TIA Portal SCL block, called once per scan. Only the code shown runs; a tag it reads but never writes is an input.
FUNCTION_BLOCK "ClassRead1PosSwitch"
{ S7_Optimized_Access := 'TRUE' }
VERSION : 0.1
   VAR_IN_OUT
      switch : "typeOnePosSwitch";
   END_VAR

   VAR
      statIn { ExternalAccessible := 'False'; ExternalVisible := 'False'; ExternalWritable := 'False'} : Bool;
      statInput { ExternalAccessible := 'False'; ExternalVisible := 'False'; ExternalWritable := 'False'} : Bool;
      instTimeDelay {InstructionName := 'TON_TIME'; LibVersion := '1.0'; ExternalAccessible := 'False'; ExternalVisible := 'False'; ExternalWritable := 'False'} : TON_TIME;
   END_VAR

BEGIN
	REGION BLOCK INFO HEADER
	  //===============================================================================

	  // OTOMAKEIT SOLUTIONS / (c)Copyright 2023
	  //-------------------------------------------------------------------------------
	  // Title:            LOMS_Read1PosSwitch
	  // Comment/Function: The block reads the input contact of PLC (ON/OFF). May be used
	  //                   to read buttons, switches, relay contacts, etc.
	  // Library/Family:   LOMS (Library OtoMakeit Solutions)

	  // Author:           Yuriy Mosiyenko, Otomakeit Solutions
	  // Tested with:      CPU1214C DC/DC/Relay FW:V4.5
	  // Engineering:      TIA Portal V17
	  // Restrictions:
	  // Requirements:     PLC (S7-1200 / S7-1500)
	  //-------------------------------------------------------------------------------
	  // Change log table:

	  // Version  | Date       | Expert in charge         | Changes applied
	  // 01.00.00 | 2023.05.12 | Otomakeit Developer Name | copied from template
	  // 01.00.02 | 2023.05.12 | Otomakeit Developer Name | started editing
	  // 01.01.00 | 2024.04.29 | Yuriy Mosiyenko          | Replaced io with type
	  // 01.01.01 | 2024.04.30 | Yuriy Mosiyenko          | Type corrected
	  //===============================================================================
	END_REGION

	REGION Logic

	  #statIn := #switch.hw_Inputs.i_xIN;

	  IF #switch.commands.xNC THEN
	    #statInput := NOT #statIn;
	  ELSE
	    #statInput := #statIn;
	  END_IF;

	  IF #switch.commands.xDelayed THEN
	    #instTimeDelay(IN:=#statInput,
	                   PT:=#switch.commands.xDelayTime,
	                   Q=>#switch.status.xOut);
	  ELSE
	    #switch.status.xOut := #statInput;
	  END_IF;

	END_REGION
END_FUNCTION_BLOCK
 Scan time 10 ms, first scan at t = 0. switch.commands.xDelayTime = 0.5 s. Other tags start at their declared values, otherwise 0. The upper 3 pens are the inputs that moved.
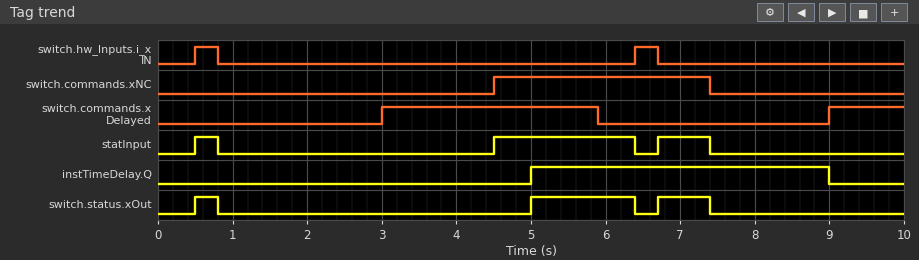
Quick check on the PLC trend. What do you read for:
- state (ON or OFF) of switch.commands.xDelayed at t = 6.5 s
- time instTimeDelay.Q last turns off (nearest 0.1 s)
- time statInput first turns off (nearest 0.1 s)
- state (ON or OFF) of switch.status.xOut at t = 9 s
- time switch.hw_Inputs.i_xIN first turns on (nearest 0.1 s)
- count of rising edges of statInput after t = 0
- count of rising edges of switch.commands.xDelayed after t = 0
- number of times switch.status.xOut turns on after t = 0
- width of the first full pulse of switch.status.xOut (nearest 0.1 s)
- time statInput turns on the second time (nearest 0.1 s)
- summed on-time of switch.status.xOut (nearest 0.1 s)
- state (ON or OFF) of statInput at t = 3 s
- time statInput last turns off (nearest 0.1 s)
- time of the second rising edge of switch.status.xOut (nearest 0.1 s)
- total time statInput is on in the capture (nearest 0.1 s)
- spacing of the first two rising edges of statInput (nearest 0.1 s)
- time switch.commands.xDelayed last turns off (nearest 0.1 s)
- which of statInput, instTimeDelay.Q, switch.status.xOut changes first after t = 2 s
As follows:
OFF
9.0 s
0.8 s
OFF
0.5 s
3
2
3
0.3 s
4.5 s
2.4 s
OFF
7.4 s
5.0 s
2.9 s
4.0 s
5.9 s
statInput
